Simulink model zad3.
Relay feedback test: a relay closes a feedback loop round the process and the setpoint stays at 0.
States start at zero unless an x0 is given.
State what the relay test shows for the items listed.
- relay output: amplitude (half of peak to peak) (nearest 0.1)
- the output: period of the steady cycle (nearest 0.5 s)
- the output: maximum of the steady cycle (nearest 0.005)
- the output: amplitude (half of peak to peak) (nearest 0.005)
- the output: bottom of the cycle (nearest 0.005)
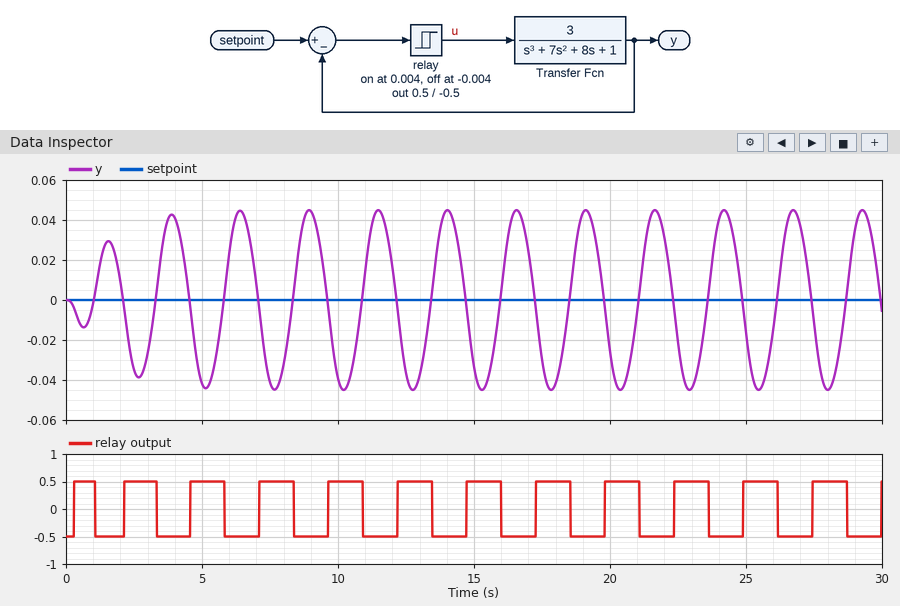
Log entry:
0.5
2.5 s
0.045
0.045
-0.045
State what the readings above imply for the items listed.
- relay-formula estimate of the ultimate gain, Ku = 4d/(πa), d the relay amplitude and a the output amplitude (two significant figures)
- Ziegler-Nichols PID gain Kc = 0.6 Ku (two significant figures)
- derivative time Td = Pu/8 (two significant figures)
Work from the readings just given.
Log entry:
14
8.4
0.31 s
